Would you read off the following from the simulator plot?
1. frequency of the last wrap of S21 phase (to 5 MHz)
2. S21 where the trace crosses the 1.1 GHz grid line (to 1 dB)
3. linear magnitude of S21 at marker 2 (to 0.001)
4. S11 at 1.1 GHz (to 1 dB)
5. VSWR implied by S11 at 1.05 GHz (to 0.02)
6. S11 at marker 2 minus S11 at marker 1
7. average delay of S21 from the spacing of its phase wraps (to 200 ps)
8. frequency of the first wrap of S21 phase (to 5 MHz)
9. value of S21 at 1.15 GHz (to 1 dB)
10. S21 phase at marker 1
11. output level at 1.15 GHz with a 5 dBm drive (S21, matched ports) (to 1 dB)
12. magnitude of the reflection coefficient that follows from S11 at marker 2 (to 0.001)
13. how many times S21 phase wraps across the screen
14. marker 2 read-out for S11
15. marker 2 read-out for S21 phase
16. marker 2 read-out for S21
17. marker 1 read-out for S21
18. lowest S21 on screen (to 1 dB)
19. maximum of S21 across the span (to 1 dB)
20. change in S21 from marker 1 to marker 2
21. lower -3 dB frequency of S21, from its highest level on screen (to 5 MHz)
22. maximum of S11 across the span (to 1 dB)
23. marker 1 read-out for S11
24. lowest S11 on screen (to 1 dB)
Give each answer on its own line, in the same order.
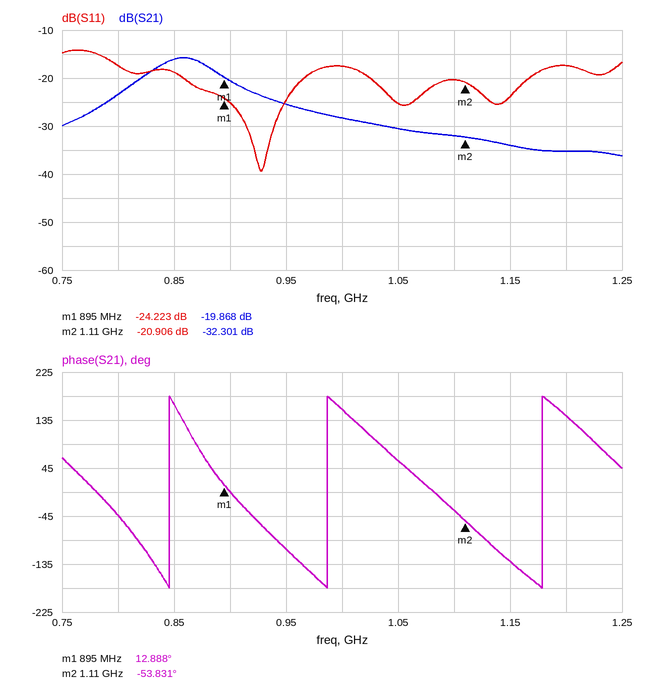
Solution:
1.180 GHz
-32 dB
0.024
-20 dB
1.12
3.317 dB
6.0 ns
845 MHz
-34 dB
12.888°
-29 dBm
0.090
3
-20.906 dB
-53.831°
-32.301 dB
-19.868 dB
-36 dB
-16 dB
-12.433 dB
830 MHz
-14 dB
-24.223 dB
-39 dB
